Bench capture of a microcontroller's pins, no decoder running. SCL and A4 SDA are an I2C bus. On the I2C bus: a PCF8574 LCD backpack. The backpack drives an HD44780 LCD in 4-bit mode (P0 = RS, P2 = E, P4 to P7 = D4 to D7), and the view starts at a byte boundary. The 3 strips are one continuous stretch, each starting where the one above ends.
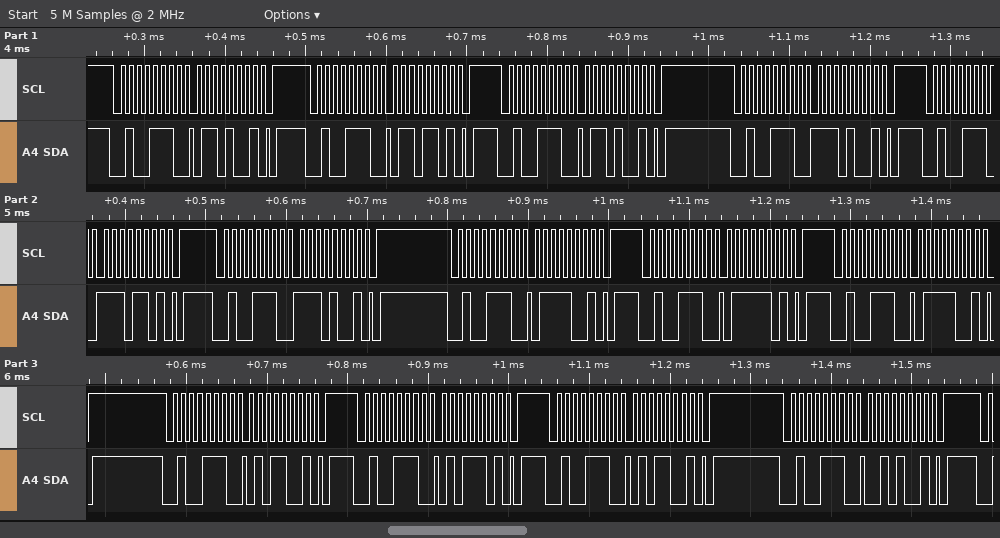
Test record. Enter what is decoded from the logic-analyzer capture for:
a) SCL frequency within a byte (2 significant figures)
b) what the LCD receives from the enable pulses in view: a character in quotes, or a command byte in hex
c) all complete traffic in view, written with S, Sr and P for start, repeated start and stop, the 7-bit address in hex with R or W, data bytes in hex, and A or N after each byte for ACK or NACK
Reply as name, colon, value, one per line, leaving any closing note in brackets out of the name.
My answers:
SCL frequency within a byte: 100 kHz
what the LCD receives from the enable pulses in view: a character in quotes, or a command byte in hex: 'n' 'u'
all complete traffic in view, written with S, Sr and P for start, repeated start and stop, the 7-bit address in hex with R or W, data bytes in hex, and A or N after each byte for ACK or NACK: S 27W A 69 A P S 27W A 6D A P S 27W A 69 A P S 27W A E9 A P S 27W A ED A P S 27W A E9 A P S 27W A 79 A P S 27W A 7D A P S 27W A 79 A P S 27W A 59 A P S 27W A 5D A P S 27W A 59 A P S 27W A 29 A P
